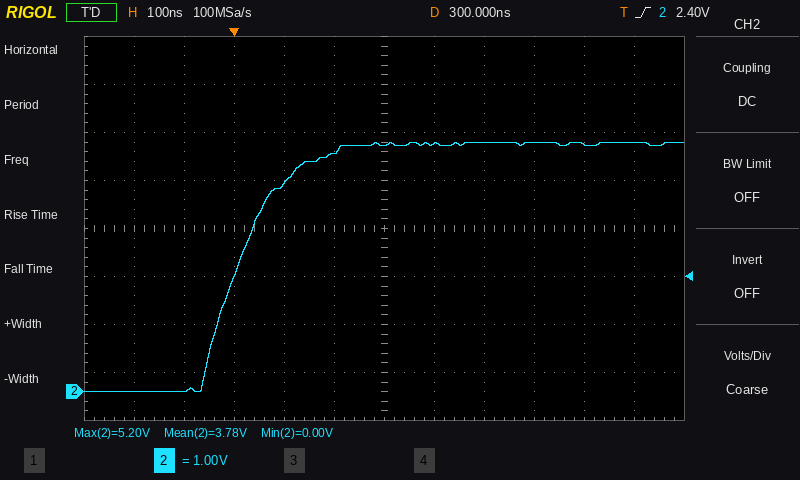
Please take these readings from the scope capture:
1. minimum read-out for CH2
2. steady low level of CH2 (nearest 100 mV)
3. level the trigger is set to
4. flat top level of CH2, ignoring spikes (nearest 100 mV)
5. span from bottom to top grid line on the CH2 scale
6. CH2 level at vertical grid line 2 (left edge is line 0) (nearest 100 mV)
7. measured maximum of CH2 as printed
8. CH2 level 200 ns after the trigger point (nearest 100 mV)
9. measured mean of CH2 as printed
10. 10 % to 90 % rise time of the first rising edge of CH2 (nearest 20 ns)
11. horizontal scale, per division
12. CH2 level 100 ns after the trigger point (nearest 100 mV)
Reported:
0.00 V
0.0 V
2.40 V
5.2 V
8 V
0.0 V
5.20 V
5.0 V
3.78 V
180 ns
100 ns
4.3 V
